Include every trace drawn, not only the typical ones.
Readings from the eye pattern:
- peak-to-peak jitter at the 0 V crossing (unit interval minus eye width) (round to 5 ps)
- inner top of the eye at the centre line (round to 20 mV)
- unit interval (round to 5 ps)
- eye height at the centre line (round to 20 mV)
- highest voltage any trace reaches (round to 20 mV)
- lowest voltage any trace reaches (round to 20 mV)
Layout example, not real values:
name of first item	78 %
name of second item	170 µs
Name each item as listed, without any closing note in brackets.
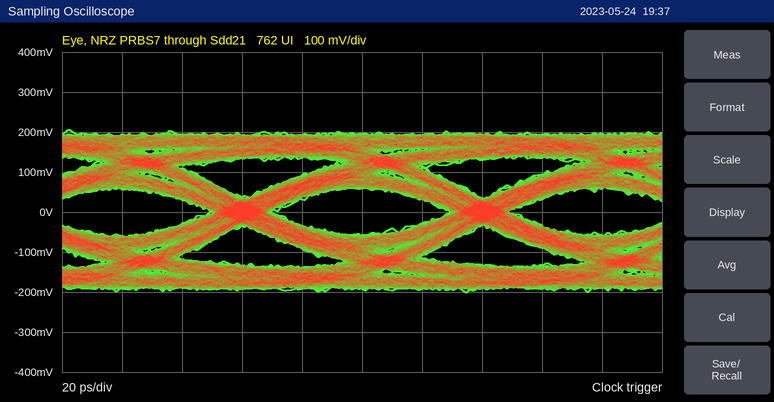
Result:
peak-to-peak jitter at the 0 V crossing (unit interval minus eye width)	20 ps
inner top of the eye at the centre line	60 mV
unit interval	80 ps
eye height at the centre line	120 mV
highest voltage any trace reaches	200 mV
lowest voltage any trace reaches	-200 mV
